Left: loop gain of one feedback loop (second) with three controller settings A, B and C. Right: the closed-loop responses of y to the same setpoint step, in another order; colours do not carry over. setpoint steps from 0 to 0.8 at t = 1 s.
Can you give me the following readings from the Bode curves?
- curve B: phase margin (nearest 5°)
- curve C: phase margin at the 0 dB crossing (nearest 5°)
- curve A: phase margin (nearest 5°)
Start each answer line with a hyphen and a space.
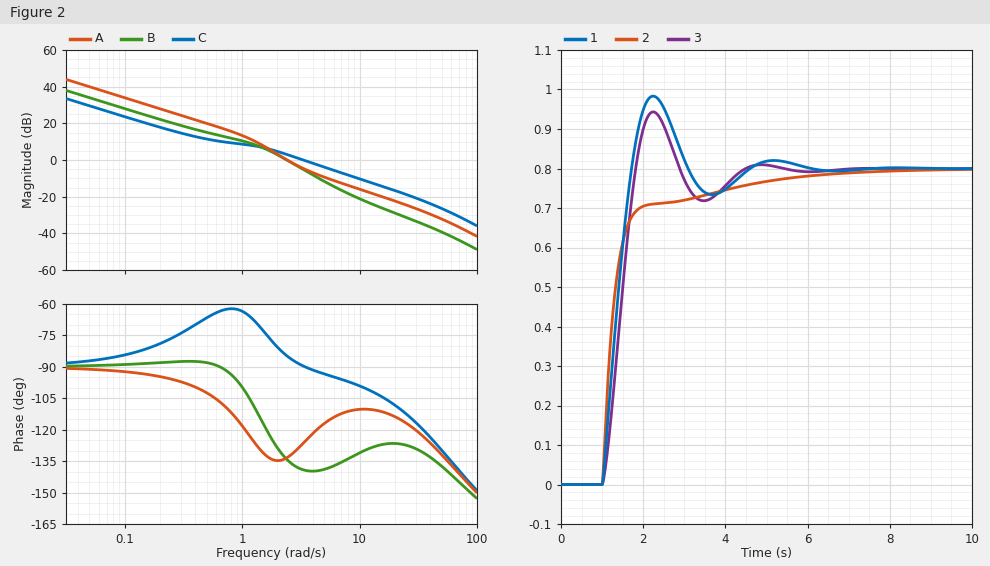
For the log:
- 45°
- 90°
- 45°
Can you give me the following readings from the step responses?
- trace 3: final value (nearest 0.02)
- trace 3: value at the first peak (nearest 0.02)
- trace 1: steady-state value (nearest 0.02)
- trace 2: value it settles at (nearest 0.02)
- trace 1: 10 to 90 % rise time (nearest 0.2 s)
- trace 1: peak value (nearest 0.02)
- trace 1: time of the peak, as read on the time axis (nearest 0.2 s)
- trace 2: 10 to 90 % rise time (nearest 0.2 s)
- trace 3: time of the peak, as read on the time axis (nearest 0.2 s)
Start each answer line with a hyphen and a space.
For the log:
- 0.80
- 0.94
- 0.80
- 0.80
- 0.6 s
- 0.98
- 2.2 s
- 2.0 s
- 2.2 s
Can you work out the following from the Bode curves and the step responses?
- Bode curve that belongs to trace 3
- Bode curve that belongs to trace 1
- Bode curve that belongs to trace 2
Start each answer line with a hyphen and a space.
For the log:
- B
- A
- C
